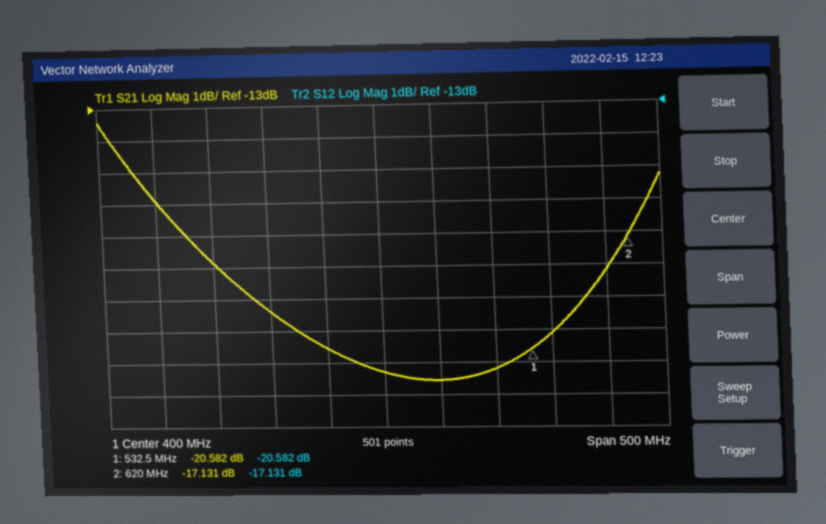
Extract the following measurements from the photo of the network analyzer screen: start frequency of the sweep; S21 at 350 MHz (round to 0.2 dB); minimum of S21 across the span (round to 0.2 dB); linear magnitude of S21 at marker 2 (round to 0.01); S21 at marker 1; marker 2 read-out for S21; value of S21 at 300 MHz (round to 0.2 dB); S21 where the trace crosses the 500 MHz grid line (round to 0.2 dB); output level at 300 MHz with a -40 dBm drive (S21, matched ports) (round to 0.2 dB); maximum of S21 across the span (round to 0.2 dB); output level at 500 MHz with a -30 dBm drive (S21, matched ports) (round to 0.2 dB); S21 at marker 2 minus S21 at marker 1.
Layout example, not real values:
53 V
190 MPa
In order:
150 MHz
-20.6 dB
-21.6 dB
0.14
-20.582 dB
-17.131 dB
-19.4 dB
-21.2 dB
-59.4 dBm
-13.4 dB
-51.2 dBm
3.451 dB
